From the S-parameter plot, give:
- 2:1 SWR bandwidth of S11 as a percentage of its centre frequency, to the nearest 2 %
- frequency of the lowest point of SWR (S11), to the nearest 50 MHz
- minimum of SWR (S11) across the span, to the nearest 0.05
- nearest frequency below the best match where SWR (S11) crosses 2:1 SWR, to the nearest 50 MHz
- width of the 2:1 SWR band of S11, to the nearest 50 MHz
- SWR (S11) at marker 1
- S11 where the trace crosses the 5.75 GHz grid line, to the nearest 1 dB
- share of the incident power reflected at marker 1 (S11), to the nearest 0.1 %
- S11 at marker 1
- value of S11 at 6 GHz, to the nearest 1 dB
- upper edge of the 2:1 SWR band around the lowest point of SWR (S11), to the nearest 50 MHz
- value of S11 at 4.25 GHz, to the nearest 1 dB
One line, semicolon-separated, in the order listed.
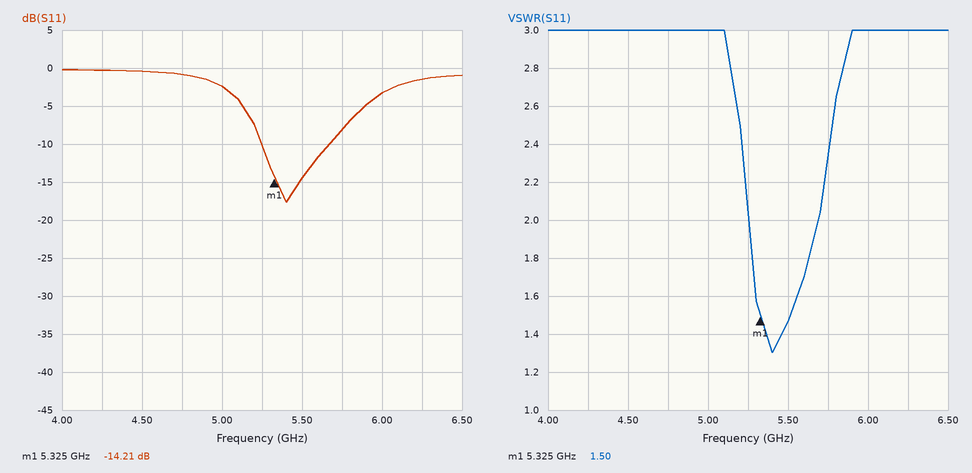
8 %; 5.40 GHz; 1.30; 5.25 GHz; 450 MHz; 1.50; -8 dB; 3.8 %; -14.21 dB; -3 dB; 5.70 GHz; 0 dB
